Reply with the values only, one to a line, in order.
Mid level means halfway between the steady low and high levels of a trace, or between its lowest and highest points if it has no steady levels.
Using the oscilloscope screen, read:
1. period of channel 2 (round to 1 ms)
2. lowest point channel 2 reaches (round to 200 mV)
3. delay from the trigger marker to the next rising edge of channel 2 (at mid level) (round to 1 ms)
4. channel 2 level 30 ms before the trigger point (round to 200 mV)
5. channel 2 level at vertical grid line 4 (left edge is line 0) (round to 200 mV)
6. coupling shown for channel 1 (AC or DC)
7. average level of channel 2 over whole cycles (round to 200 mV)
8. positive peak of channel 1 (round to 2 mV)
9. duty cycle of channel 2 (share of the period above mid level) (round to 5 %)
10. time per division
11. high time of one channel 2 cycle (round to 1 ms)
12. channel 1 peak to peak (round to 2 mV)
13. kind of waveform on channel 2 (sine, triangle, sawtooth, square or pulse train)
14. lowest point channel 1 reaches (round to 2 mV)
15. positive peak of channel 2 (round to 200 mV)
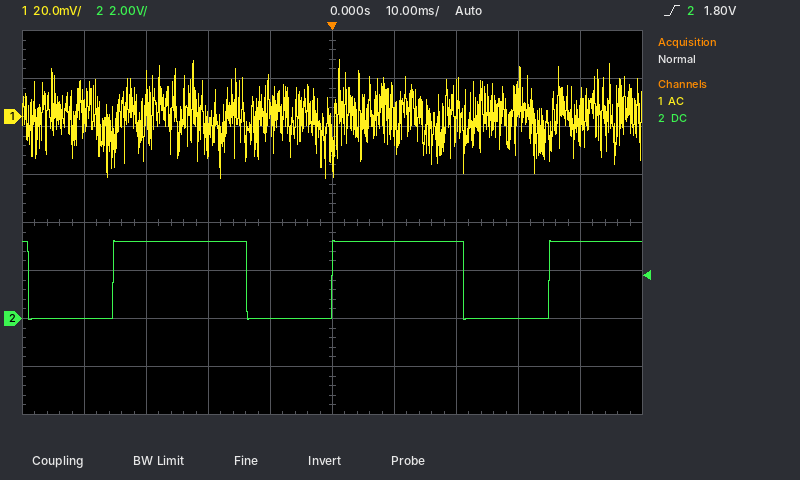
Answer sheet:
35 ms
0.0 V
35 ms
3.2 V
0.0 V
AC
2.0 V
24 mV
60 %
10 ms
21 ms
50 mV
pulse train
-26 mV
3.2 V
